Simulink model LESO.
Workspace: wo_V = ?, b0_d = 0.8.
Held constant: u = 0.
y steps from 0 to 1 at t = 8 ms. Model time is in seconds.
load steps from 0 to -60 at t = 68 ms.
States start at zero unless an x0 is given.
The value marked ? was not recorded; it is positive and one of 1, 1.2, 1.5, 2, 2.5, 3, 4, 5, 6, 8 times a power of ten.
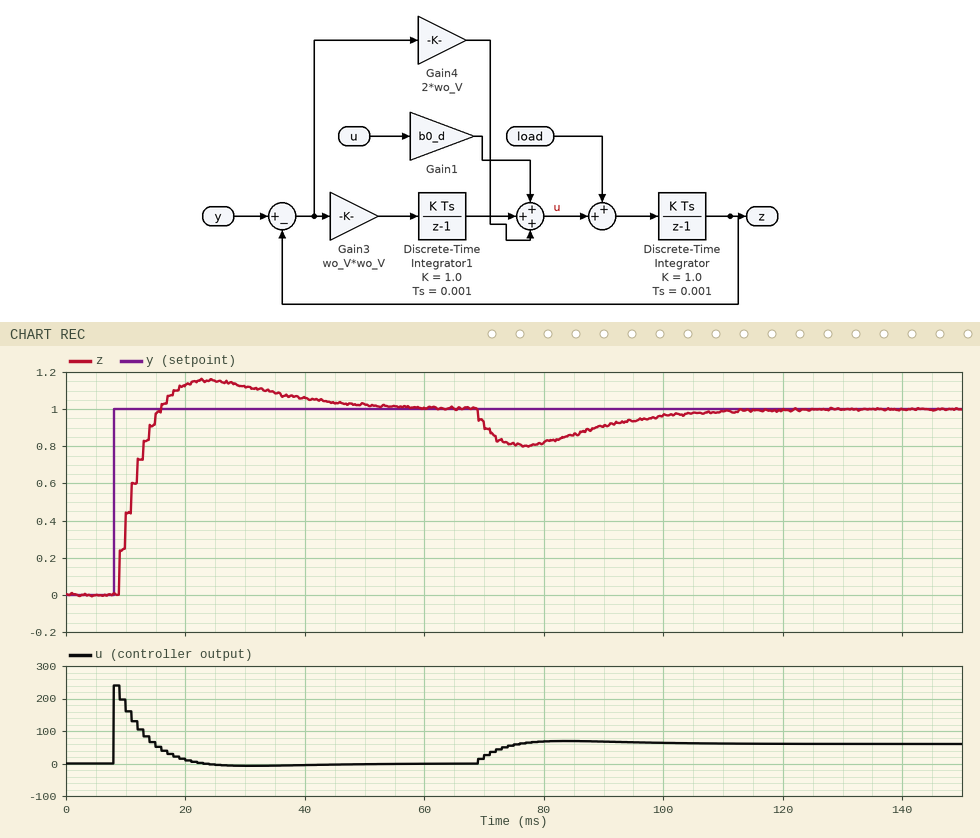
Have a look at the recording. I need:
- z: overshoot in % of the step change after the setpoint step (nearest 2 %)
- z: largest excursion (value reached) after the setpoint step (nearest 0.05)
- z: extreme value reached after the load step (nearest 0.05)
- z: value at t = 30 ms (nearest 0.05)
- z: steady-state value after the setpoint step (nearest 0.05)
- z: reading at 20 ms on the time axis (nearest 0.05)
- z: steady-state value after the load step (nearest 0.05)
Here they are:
16 %
1.15
0.80
1.10
1.00
1.15
1.00
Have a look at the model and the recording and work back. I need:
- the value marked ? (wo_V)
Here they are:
120
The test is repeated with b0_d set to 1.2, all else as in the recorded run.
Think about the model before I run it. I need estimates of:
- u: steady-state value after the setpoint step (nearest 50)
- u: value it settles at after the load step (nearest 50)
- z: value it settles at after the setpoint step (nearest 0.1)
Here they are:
0
50
1.0
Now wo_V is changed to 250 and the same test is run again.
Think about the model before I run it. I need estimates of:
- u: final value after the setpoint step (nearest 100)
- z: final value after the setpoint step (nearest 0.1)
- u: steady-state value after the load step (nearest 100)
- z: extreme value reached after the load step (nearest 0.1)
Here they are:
0
1.0
100
0.9
